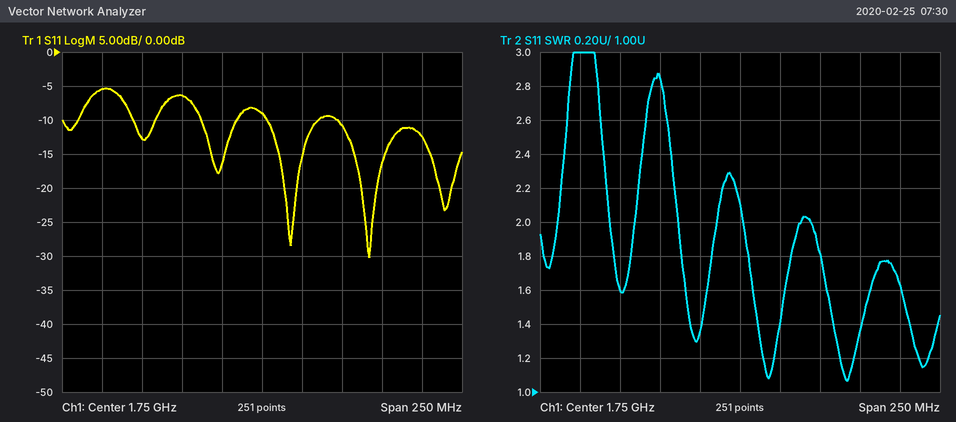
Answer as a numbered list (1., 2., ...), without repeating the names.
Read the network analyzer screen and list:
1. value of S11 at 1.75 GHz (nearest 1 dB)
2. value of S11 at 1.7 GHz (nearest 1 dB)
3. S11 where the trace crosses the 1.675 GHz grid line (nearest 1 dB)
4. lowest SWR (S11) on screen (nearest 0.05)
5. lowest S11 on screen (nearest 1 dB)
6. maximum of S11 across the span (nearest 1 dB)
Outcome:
1. -9 dB
2. -6 dB
3. -13 dB
4. 1.05
5. -30 dB
6. -5 dB
